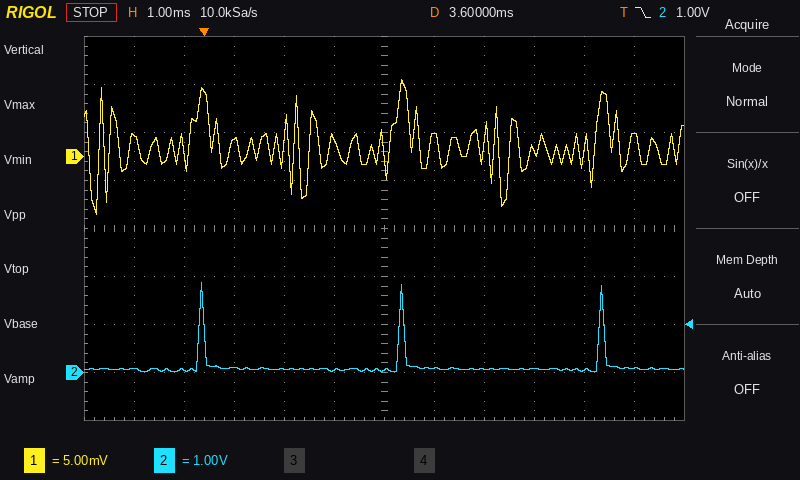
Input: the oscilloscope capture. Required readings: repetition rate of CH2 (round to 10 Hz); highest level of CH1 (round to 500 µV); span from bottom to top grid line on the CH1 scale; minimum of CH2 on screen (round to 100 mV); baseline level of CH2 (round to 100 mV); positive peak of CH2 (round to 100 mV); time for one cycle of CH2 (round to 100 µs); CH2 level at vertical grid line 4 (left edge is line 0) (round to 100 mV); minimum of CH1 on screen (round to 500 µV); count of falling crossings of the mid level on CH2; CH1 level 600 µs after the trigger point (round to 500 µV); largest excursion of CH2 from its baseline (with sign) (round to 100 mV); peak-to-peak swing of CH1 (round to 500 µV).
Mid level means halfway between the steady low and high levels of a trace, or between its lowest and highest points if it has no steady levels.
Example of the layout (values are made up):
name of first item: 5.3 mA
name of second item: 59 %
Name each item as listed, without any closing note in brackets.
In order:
repetition rate of CH2: 250 Hz
highest level of CH1: 8.0 mV
span from bottom to top grid line on the CH1 scale: 40 mV
minimum of CH2 on screen: 0.0 V
baseline level of CH2: 100 mV
positive peak of CH2: 1.9 V
time for one cycle of CH2: 4.0 ms
CH2 level at vertical grid line 4 (left edge is line 0): 100 mV
minimum of CH1 on screen: -6.0 mV
count of falling crossings of the mid level on CH2: 3
CH1 level 600 µs after the trigger point: 1.5 mV
largest excursion of CH2 from its baseline (with sign): +1.8 V
peak-to-peak swing of CH1: 14.0 mV
